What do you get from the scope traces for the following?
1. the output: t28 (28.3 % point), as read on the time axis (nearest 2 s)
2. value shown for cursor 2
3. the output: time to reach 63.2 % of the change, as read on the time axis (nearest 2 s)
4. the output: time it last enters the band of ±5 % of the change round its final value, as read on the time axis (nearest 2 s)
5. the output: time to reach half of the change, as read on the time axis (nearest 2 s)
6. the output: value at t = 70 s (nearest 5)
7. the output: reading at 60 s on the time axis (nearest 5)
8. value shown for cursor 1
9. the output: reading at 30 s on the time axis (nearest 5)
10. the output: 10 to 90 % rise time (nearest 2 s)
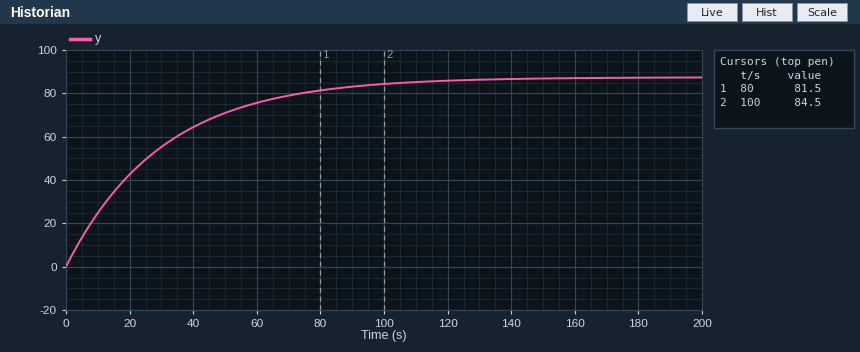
10 s
84.5
30 s
90 s
20 s
80
75
81.5
55
66 s
